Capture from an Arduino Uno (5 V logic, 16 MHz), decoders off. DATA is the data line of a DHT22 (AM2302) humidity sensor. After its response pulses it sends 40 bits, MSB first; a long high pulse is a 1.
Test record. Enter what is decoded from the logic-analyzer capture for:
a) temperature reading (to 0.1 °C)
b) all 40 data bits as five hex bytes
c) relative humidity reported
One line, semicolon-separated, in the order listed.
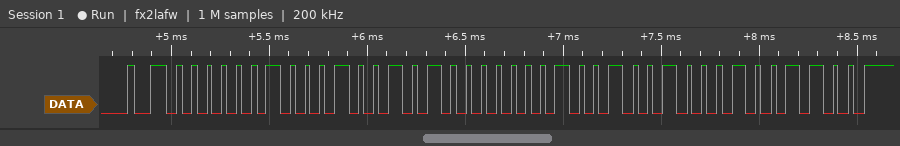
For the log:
29.2 °C; 02 25 01 24 4C; 54.9 %
